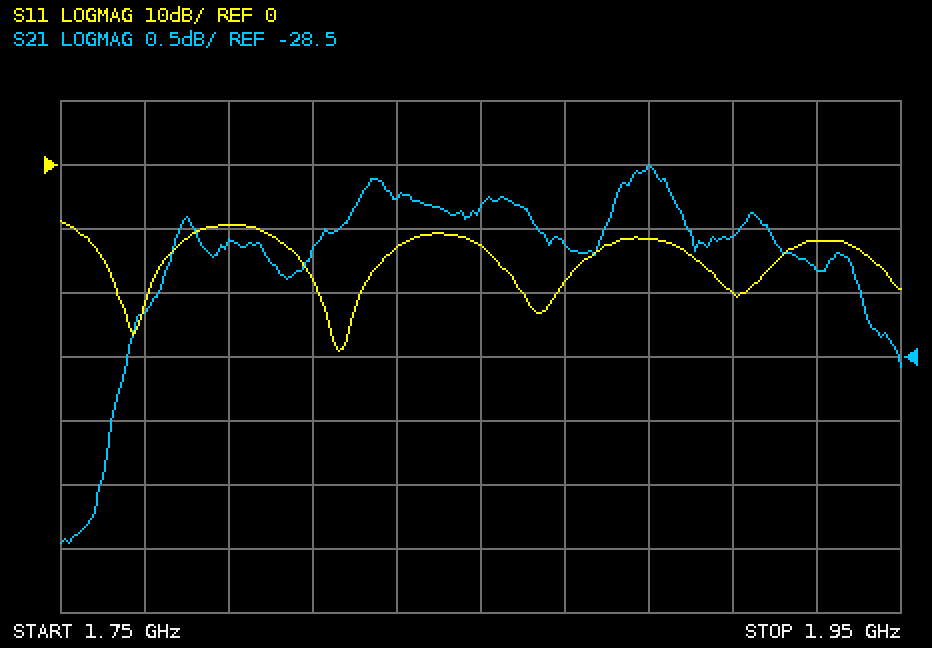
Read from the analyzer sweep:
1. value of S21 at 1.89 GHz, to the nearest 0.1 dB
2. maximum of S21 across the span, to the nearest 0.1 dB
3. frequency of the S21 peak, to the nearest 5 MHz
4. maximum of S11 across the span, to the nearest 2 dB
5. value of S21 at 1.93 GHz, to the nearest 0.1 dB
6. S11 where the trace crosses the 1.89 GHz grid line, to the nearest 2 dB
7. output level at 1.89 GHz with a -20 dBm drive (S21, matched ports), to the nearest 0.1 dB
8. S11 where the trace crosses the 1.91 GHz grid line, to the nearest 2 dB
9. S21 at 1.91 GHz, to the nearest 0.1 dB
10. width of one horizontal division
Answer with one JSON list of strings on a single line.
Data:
["-27.0 dB", "-27.0 dB", "1.890 GHz", "-8 dB", "-27.8 dB", "-12 dB", "-47.0 dBm", "-20 dB", "-27.6 dB", "20 MHz"]
